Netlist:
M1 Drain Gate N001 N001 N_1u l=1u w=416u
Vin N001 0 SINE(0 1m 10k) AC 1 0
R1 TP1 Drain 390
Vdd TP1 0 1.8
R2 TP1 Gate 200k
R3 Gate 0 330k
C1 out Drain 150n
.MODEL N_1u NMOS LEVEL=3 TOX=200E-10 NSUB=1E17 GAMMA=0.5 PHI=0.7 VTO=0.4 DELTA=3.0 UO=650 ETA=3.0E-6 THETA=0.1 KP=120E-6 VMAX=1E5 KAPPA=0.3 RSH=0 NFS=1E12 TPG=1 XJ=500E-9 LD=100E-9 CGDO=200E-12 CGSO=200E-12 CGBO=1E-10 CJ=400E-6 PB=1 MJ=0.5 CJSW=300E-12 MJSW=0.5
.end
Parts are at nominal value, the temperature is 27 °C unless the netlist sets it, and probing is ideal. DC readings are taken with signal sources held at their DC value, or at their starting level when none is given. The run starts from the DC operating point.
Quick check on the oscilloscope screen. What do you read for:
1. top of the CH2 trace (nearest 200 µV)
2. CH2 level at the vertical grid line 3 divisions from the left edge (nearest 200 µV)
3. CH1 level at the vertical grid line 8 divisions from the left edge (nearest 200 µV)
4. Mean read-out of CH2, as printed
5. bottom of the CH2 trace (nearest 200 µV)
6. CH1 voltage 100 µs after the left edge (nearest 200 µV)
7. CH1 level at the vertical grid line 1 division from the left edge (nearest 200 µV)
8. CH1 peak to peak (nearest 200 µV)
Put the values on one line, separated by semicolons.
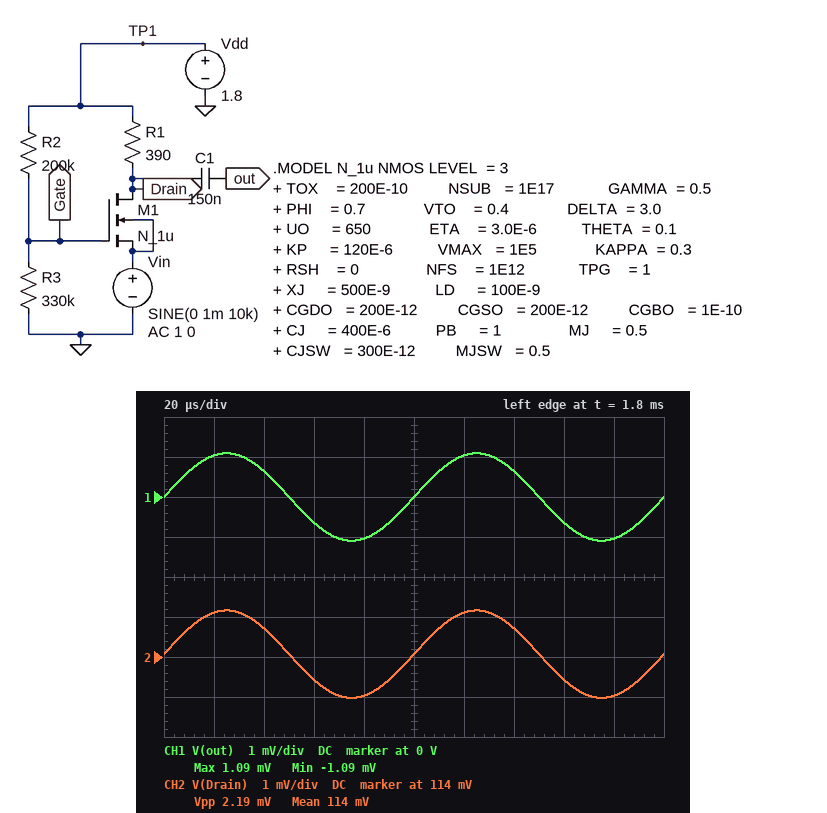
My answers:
115.2 mV; 113.4 mV; -600 µV; 114 mV; 113.0 mV; 0 V; 1.0 mV; 2.2 mV
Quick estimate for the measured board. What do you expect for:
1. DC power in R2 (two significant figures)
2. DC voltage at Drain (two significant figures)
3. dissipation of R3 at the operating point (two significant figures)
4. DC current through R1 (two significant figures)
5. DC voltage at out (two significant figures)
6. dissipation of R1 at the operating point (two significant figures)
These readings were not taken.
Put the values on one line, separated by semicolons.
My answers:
2.3 µW; 110 mV; 3.8 µW; 4.3 mA; 110 mV; 7.3 mW
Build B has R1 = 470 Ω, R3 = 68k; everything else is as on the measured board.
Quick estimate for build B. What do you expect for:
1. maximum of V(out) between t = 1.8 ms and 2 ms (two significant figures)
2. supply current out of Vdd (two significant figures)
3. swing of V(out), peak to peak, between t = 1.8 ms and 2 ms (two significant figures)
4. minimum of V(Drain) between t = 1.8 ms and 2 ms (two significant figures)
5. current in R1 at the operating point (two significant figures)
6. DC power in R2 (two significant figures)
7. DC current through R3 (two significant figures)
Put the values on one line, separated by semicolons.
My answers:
2.7 mV; 340 µA; 5.4 mV; 1.6 V; 330 µA; 9.0 µW; 6.7 µA
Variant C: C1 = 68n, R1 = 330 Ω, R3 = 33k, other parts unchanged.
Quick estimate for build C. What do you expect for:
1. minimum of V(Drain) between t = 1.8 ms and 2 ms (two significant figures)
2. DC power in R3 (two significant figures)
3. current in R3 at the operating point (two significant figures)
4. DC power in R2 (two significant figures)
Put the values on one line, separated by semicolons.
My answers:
1.8 V; 2.0 µW; 7.7 µA; 12 µW
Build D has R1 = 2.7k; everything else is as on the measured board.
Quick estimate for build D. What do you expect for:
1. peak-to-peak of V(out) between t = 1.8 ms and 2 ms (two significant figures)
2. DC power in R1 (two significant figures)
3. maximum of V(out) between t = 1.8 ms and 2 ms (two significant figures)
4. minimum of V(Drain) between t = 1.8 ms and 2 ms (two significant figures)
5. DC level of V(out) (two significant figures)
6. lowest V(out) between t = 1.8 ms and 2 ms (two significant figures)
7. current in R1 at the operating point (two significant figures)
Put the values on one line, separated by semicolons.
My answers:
2.0 mV; 1.2 mW; 1.0 mV; 14 mV; 15 mV; -1.0 mV; 660 µA
